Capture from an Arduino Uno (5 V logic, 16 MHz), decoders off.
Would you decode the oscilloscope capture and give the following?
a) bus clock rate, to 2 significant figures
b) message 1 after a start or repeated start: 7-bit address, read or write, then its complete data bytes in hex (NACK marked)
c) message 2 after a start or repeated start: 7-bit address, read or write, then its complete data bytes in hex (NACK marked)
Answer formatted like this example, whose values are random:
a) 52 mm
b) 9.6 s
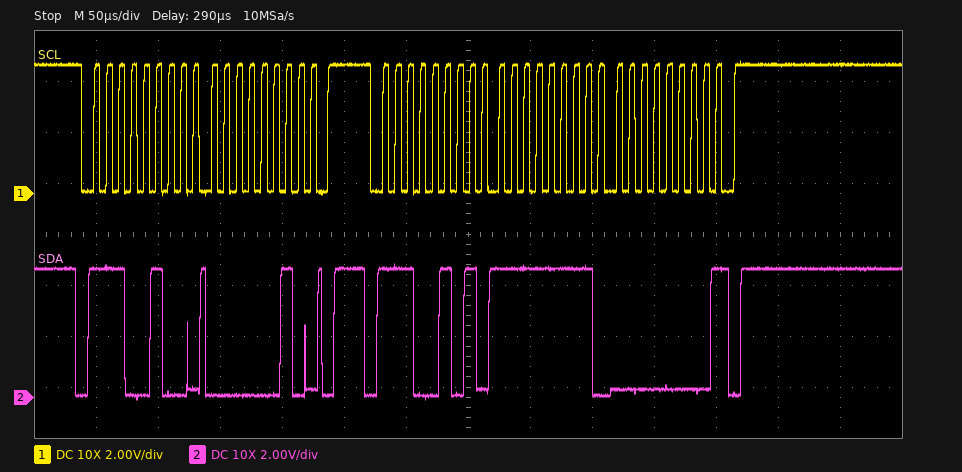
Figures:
a) 100 kHz
b) 0x72 write: 02
c) 0x72 read: FF 00 NACK
